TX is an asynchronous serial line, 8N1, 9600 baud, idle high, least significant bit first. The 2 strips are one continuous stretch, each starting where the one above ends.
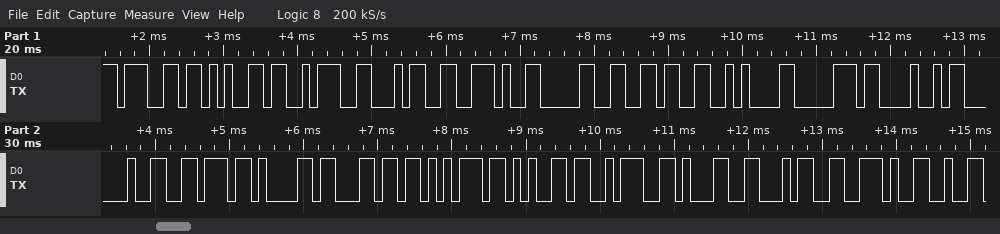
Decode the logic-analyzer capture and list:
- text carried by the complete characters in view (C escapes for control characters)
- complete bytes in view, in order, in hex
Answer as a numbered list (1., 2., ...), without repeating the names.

1. "ge:4.06\npH value:14."
2. 67 65 3A 34 2E 30 36 0A 70 48 20 76 61 6C 75 65 3A 31 34 2E
